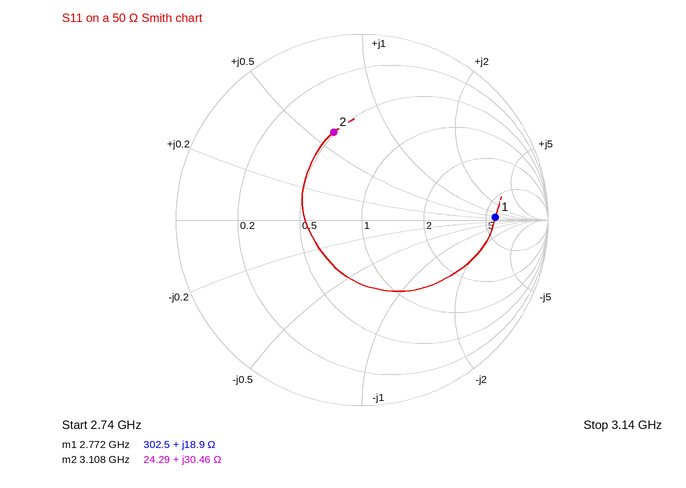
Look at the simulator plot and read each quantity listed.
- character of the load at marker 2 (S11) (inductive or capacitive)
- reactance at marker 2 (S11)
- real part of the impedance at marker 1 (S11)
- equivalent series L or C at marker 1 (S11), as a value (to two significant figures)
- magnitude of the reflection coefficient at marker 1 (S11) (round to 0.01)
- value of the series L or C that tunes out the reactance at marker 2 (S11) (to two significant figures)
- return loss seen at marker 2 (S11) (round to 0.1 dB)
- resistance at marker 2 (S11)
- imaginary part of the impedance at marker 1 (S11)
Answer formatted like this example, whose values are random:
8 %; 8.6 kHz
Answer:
inductive; +30.46 Ω; 302.5 Ω; 1.1 nH; 0.72; 1.7 pF; 6.1 dB; 24.29 Ω; +18.9 Ω
